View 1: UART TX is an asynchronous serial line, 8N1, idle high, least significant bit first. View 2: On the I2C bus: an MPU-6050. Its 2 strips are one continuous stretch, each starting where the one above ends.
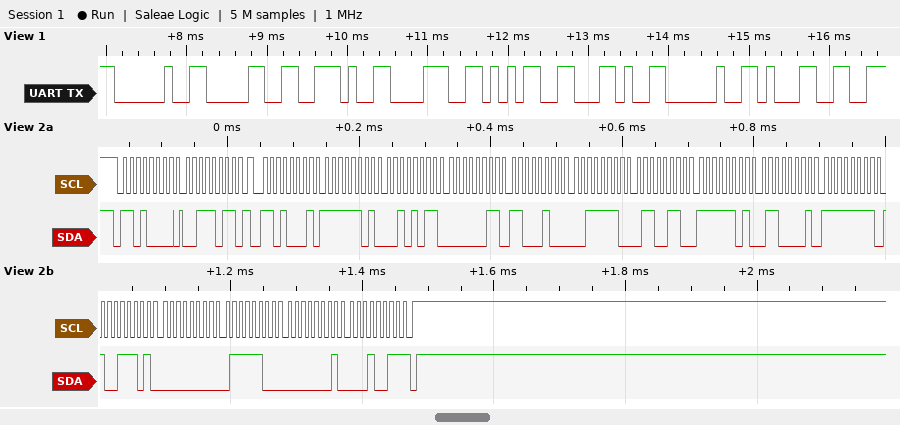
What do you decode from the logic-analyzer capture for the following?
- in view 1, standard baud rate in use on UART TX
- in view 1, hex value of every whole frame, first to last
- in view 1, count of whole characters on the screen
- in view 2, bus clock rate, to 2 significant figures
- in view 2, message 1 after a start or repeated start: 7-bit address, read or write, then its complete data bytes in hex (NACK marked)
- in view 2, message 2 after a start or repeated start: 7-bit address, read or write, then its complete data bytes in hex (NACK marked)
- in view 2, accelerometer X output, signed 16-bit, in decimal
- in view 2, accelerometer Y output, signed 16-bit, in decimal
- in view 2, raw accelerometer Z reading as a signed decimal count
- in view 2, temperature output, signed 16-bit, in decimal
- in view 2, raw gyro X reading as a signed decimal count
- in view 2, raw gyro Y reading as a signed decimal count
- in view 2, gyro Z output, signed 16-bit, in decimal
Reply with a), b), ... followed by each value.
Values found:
a) 9600 baud
b) 0x20 0x30 0x2E 0x38 0x35 0x2C 0x20 0x31
c) 8
d) 100 kHz
e) 0x68 write: 3B
f) 0x68 read: FD 2B 03 C4 3E 66 FD 61 FF 9D 00 7C 01 13 NACK
g) -725
h) 964
i) 15974
j) -671
k) -99
l) 124
m) 275
